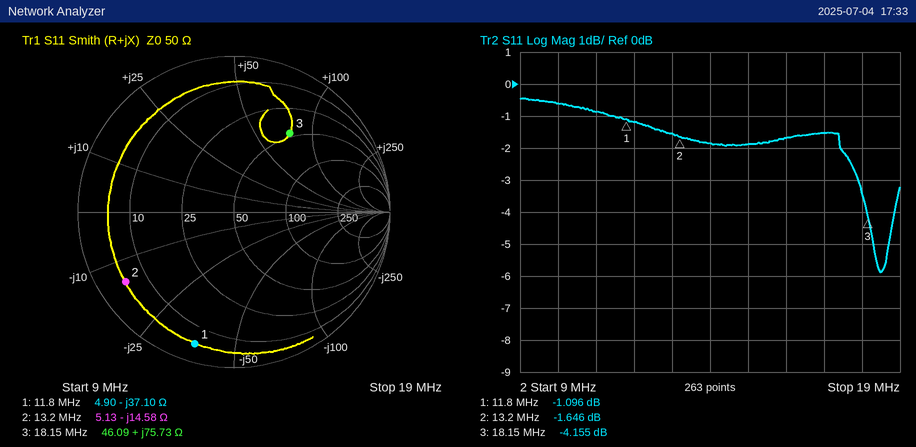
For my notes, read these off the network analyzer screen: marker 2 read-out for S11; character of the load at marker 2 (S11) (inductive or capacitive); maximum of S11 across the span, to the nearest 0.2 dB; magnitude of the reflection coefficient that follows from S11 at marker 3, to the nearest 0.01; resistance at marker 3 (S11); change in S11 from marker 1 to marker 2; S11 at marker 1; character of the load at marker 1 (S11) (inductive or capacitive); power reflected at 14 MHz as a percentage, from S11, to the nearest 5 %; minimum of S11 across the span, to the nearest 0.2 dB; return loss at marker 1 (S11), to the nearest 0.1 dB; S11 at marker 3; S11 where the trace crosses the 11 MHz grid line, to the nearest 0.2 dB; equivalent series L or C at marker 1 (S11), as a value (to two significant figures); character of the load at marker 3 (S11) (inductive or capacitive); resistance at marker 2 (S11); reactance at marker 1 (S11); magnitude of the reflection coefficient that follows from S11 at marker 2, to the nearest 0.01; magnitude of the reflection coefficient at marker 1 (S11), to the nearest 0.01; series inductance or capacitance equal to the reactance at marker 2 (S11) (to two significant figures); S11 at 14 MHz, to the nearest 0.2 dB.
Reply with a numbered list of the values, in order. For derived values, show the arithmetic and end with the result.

1. -1.646 dB
2. capacitive
3. -0.4 dB
4. 10^(-4.155/20) ≈ 0.62
5. 46.09 Ω
6. -1.646 − (-1.096) = -0.550 dB
7. -1.096 dB
8. capacitive
9. 10^(-1.8/10) ≈ 66.1 %, so 65 % to the nearest 5 %
10. -5.8 dB
11. 1.1 dB
12. -4.155 dB
13. -0.8 dB
14. C = 1/(2π × 11.8 MHz × 37.1 Ω) ≈ 364 pF, so 360 pF to two significant figures
15. inductive
16. 5.13 Ω
17. -37.10 Ω
18. 10^(-1.646/20) ≈ 0.83
19. 10^(-1.096/20) ≈ 0.88
20. C = 1/(2π × 13.2 MHz × 14.58 Ω) ≈ 827 pF, so 830 pF to two significant figures
21. -1.8 dB
